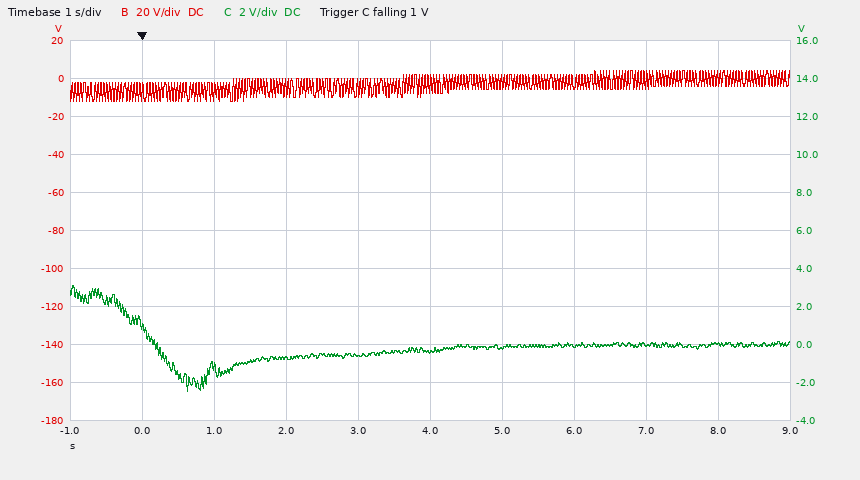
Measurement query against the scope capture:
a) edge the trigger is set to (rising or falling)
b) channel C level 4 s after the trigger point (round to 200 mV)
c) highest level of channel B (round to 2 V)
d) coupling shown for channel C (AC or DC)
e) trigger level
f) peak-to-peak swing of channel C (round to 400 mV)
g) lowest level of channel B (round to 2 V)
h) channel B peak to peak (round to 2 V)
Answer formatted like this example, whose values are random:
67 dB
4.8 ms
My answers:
falling
-400 mV
4 V
DC
1 V
5.6 V
-12 V
16 V
